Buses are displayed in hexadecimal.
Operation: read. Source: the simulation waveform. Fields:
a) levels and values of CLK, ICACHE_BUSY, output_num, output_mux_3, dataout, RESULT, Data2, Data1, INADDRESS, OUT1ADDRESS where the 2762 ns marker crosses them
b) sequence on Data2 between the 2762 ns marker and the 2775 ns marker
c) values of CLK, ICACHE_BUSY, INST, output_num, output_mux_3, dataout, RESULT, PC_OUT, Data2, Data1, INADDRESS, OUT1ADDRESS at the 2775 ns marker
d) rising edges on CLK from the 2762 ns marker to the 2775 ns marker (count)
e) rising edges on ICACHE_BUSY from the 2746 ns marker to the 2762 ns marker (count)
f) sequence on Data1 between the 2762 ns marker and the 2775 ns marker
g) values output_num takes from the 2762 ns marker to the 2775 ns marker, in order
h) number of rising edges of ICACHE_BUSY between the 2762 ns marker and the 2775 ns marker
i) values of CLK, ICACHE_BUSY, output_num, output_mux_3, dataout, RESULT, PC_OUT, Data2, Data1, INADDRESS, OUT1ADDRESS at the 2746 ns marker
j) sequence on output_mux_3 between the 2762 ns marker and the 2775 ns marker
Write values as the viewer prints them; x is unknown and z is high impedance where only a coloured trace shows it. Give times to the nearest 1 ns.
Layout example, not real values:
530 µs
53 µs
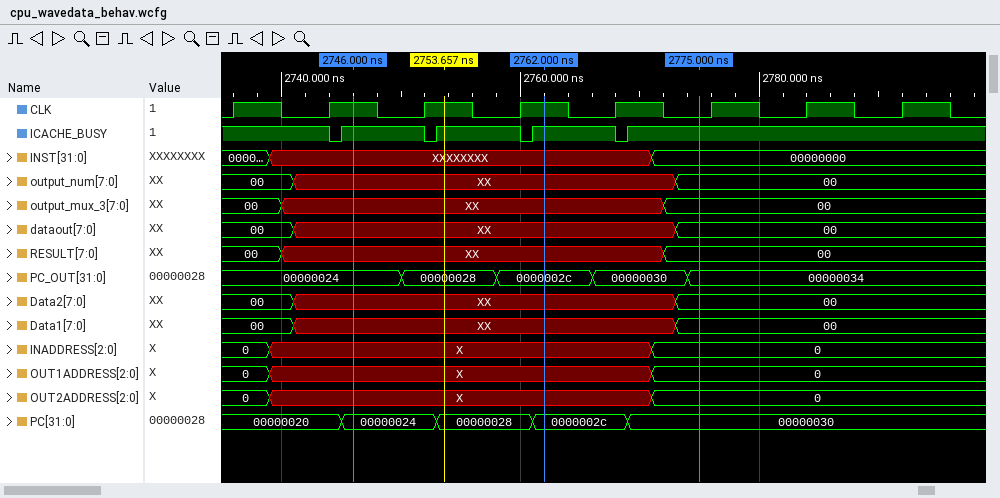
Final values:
CLK=1, ICACHE_BUSY=1, output_num=XX, output_mux_3=XX, dataout=XX, RESULT=XX, Data2=XX, Data1=XX, INADDRESS=X, OUT1ADDRESS=X
XX, 00
CLK=0, ICACHE_BUSY=1, INST=00000000, output_num=00, output_mux_3=00, dataout=00, RESULT=00, PC_OUT=00000034, Data2=00, Data1=00, INADDRESS=0, OUT1ADDRESS=0
1
2
XX, 00
XX, 00
1
CLK=1, ICACHE_BUSY=1, output_num=XX, output_mux_3=XX, dataout=XX, RESULT=XX, PC_OUT=00000024, Data2=XX, Data1=XX, INADDRESS=X, OUT1ADDRESS=X
XX, 00
